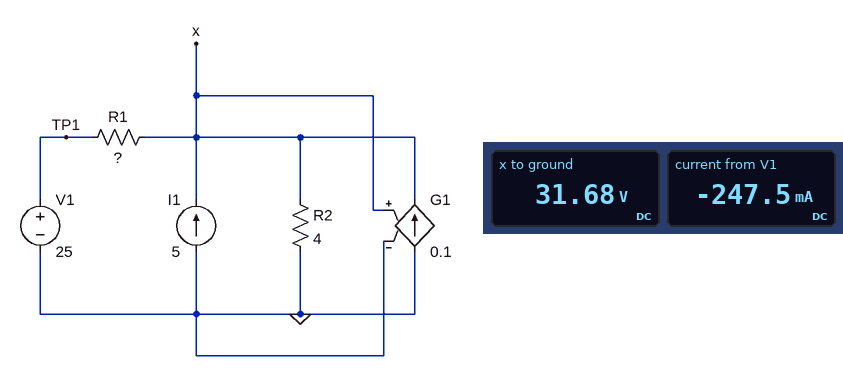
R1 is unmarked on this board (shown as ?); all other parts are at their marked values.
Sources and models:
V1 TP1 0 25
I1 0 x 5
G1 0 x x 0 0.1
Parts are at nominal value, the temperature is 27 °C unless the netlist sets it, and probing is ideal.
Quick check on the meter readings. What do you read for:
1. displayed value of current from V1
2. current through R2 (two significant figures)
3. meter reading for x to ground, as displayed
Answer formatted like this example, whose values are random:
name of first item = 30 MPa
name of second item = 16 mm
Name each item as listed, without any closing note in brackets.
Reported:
displayed value of current from V1 = -247.5 mA
current through R2 = 7.9 A
meter reading for x to ground, as displayed = 31.68 V
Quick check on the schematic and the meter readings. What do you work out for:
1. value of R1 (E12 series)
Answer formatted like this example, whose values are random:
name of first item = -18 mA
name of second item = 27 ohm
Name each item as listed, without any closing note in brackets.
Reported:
value of R1 = 27 Ω
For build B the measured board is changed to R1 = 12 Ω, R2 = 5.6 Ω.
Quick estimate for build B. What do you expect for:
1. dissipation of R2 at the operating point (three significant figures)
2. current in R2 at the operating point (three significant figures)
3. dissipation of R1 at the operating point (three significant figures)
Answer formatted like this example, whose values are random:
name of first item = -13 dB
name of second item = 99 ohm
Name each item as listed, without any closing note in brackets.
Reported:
dissipation of R2 at the operating point = 342 W
current in R2 at the operating point = 7.81 A
dissipation of R1 at the operating point = 29.3 W
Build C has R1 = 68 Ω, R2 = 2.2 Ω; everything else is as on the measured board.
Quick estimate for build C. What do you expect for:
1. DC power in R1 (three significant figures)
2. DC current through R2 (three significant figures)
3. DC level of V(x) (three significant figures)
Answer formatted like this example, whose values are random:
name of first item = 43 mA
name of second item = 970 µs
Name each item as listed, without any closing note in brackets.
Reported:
DC power in R1 = 1.61 W
DC current through R2 = 6.61 A
DC level of V(x) = 14.5 V
